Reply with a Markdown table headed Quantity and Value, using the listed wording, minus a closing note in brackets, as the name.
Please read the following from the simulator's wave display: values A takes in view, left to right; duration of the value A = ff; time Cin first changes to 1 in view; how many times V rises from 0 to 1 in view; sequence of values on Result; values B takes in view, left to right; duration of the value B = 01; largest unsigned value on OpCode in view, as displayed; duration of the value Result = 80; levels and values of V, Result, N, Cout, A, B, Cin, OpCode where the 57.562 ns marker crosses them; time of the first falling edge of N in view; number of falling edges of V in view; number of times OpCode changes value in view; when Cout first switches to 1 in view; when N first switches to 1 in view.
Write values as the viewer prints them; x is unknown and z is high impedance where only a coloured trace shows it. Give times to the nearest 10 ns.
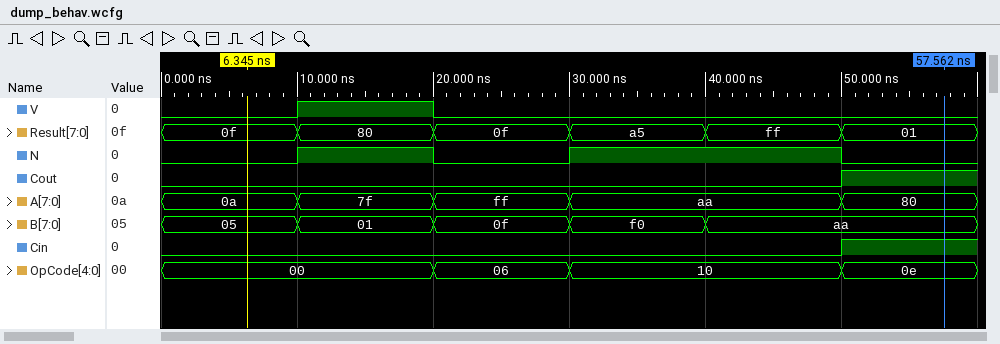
| Quantity | Value |
|---|---|
| values A takes in view, left to right | 0a, 7f, ff, aa, 80 |
| duration of the value A = ff | 10 ns |
| time Cin first changes to 1 in view | 50 ns |
| how many times V rises from 0 to 1 in view | 1 |
| sequence of values on Result | 0f, 80, 0f, a5, ff, 01 |
| values B takes in view, left to right | 05, 01, 0f, f0, aa |
| duration of the value B = 01 | 10 ns |
| largest unsigned value on OpCode in view, as displayed | 10 |
| duration of the value Result = 80 | 10 ns |
| levels and values of V, Result, N, Cout, A, B, Cin, OpCode where the 57.562 ns marker crosses them | V=0, Result=01, N=0, Cout=1, A=80, B=aa, Cin=1, OpCode=0e |
| time of the first falling edge of N in view | 20 ns |
| number of falling edges of V in view | 1 |
| number of times OpCode changes value in view | 3 |
| when Cout first switches to 1 in view | 50 ns |
| when N first switches to 1 in view | 10 ns |
